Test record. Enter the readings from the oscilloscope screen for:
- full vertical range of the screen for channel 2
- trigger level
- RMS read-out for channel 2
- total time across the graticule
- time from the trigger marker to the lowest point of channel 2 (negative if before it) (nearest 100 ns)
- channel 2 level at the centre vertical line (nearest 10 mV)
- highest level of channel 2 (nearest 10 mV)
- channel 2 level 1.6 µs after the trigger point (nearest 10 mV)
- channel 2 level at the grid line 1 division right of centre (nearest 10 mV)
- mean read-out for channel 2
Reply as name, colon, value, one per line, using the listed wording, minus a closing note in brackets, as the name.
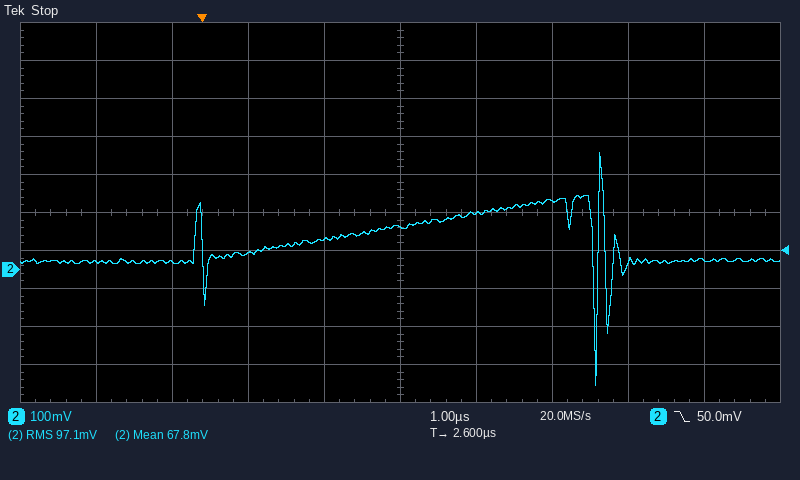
full vertical range of the screen for channel 2: 1 V
trigger level: 50.0 mV
RMS read-out for channel 2: 97.1 mV
total time across the graticule: 10 µs
time from the trigger marker to the lowest point of channel 2 (negative if before it): +5.2 µs
channel 2 level at the centre vertical line: 110 mV
highest level of channel 2: 310 mV
channel 2 level 1.6 µs after the trigger point: 80 mV
channel 2 level at the grid line 1 division right of centre: 150 mV
mean read-out for channel 2: 67.8 mV
